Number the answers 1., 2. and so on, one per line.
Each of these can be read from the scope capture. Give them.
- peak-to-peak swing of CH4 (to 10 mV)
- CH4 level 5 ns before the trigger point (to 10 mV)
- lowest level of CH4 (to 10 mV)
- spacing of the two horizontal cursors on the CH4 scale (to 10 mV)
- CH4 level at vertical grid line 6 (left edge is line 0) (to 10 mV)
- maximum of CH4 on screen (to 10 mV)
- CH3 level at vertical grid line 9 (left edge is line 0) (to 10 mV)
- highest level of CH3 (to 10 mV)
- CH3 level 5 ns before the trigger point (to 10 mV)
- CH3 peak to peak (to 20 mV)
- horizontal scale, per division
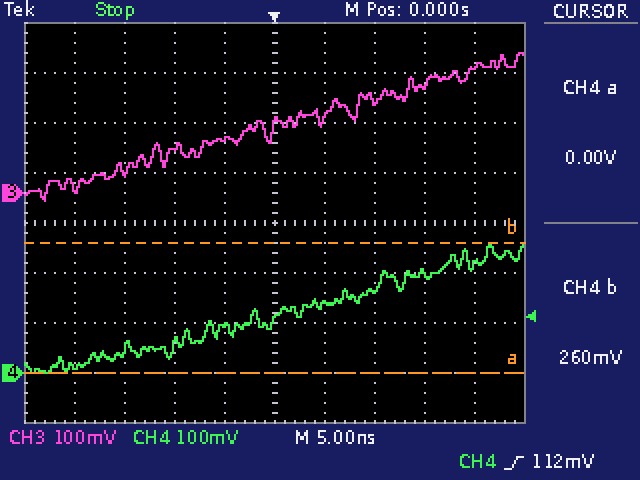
1. 260 mV
2. 100 mV
3. 0 mV
4. 260 mV
5. 140 mV
6. 260 mV
7. 250 mV
8. 280 mV
9. 110 mV
10. 300 mV
11. 5 ns
